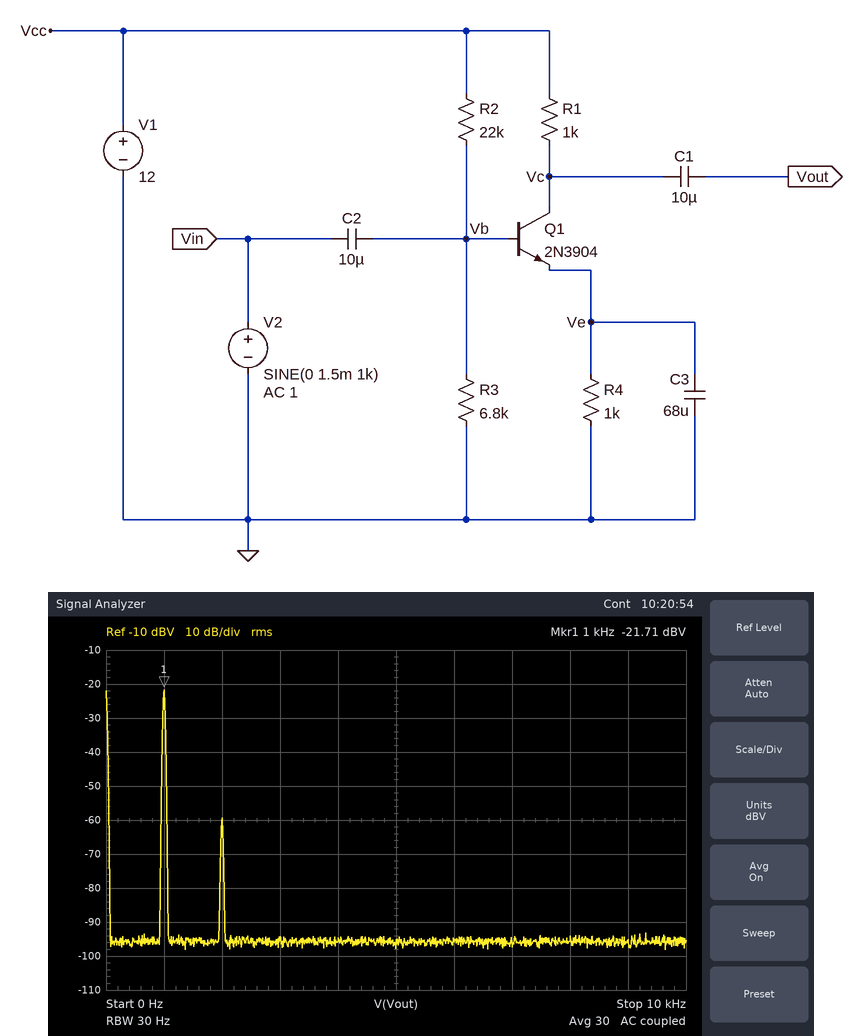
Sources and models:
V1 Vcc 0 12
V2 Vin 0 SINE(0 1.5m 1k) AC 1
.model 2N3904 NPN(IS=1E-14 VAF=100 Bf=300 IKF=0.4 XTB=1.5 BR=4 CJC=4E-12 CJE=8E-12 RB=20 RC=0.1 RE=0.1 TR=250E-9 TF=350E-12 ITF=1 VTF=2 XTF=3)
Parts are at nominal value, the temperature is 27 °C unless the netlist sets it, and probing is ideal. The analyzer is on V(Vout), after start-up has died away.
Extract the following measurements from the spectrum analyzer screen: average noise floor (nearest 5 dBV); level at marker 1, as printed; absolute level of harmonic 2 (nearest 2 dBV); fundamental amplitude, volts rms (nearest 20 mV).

-95 dBV
-21.71 dBV
-60 dBV
80 mV
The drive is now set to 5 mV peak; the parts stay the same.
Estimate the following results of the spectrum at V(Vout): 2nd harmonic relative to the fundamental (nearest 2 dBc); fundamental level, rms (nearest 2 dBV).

-28 dBc
-12 dBV
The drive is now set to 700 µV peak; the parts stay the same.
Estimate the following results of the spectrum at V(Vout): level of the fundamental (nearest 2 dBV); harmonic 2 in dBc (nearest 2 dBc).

-28 dBV
-44 dBc
